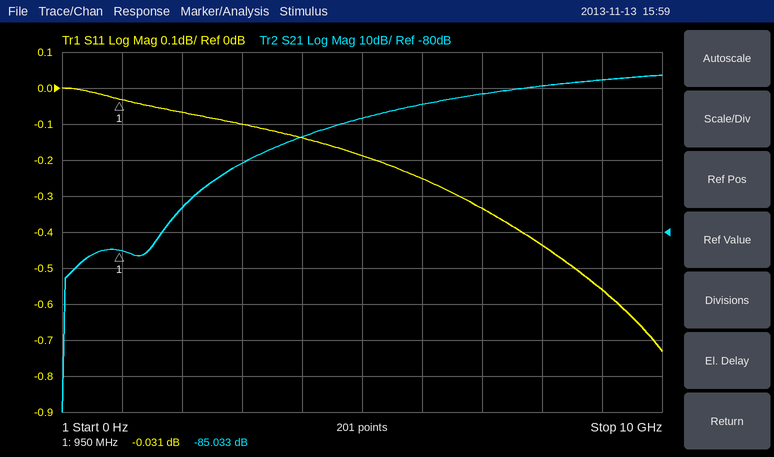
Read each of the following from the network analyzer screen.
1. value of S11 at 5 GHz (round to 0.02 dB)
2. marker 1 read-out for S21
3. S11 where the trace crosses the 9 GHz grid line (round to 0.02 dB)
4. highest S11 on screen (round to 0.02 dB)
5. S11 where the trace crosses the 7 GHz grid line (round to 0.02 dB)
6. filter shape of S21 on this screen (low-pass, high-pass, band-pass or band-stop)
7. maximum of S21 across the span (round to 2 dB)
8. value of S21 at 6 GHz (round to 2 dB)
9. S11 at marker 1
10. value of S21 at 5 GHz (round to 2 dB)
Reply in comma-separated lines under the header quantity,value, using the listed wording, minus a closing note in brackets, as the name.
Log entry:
quantity,value
value of S11 at 5 GHz,-0.18 dB
marker 1 read-out for S21,-85.033 dB
S11 where the trace crosses the 9 GHz grid line,-0.56 dB
highest S11 on screen,0.00 dB
S11 where the trace crosses the 7 GHz grid line,-0.34 dB
filter shape of S21 on this screen,high-pass
maximum of S21 across the span,-36 dB
value of S21 at 6 GHz,-44 dB
S11 at marker 1,-0.031 dB
value of S21 at 5 GHz,-48 dB
